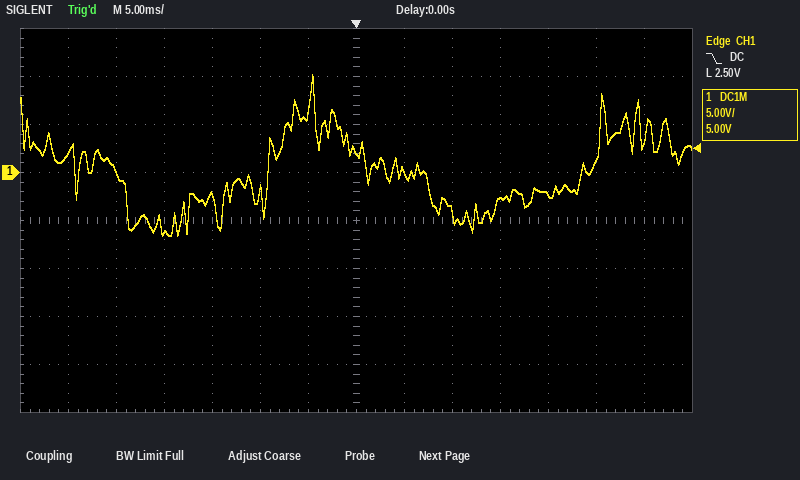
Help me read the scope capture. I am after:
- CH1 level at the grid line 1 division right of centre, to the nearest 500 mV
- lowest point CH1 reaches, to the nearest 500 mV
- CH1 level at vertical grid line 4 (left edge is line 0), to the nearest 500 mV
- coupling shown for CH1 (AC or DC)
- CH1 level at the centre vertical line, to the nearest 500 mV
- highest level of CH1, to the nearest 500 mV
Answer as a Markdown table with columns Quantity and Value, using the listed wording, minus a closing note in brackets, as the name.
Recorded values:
| Quantity | Value |
|---|---|
| CH1 level at the grid line 1 division right of centre, to the nearest 500 mV | 0.0 V |
| lowest point CH1 reaches, to the nearest 500 mV | -6.5 V |
| CH1 level at vertical grid line 4 (left edge is line 0), to the nearest 500 mV | -2.5 V |
| coupling shown for CH1 | DC |
| CH1 level at the centre vertical line, to the nearest 500 mV | 2.0 V |
| highest level of CH1, to the nearest 500 mV | 10.0 V |
